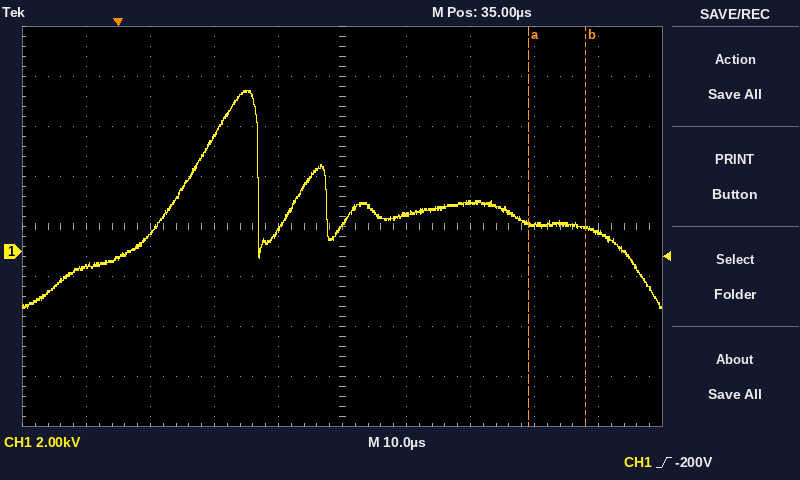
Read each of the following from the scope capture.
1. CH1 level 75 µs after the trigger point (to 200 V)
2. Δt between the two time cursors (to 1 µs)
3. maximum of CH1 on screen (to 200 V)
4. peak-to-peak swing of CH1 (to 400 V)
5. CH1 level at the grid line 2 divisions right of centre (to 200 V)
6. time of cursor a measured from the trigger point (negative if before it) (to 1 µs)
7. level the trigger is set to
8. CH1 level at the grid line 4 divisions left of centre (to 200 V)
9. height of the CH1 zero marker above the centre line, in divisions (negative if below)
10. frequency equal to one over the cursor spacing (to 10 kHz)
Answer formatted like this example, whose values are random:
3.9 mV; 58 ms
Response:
800 V; 9 µs; 6.4 kV; 8.8 kV; 2.0 kV; +64 µs; -200 V; -600 V; -0.5 div; 110 kHz
